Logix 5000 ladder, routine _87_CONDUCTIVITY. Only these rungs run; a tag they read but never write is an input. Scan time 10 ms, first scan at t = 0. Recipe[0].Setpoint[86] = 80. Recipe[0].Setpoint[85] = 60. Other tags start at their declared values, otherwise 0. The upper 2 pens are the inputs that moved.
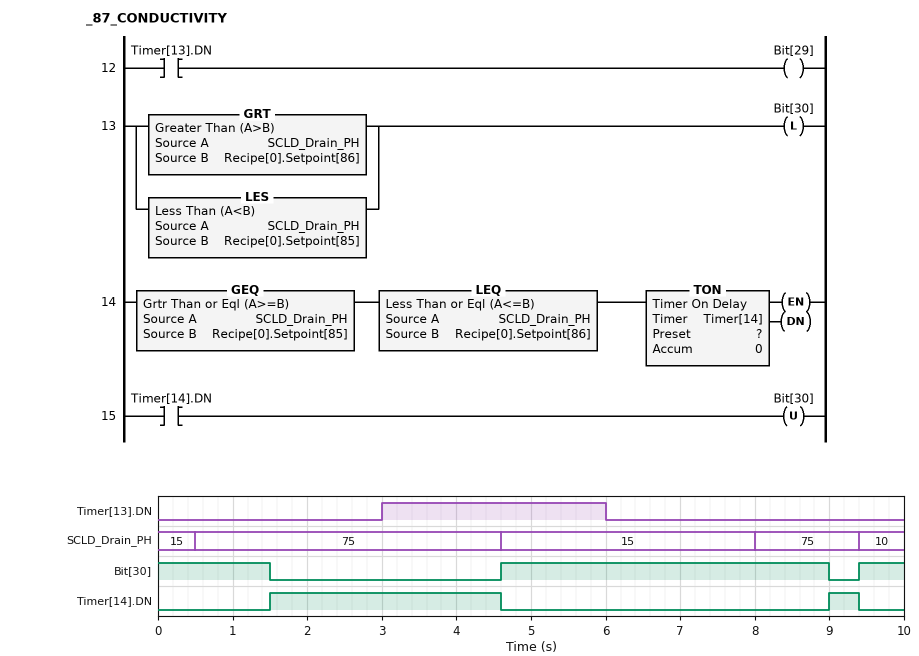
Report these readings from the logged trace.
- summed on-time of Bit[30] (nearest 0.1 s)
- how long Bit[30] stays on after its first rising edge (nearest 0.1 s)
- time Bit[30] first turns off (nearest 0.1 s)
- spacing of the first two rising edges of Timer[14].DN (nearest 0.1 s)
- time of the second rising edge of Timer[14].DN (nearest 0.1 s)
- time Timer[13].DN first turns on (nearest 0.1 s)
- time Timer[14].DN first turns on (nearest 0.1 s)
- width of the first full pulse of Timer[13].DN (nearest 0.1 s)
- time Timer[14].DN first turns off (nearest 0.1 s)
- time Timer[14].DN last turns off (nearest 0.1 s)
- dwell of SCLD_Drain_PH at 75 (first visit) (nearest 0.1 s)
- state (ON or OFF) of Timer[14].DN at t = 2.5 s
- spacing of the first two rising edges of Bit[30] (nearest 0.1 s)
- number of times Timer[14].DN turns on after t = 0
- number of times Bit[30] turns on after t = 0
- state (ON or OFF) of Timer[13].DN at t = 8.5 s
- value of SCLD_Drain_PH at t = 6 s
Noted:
6.5 s
4.4 s
1.5 s
7.5 s
9.0 s
3.0 s
1.5 s
3.0 s
4.6 s
9.4 s
4.1 s
ON
4.8 s
2
2
OFF
15
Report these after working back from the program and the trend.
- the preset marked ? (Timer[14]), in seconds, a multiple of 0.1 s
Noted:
1.0 s
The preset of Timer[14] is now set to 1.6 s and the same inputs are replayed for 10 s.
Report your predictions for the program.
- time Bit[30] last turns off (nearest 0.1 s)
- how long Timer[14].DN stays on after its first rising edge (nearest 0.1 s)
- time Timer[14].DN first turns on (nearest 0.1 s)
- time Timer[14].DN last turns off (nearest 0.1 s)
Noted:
2.1 s
2.5 s
2.1 s
4.6 s
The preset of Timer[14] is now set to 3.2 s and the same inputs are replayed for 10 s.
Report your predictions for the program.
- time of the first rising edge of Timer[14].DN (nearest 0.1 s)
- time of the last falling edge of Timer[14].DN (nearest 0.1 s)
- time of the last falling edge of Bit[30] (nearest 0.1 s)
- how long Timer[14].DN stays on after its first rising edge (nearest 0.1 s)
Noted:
3.7 s
4.6 s
3.7 s
0.9 s
